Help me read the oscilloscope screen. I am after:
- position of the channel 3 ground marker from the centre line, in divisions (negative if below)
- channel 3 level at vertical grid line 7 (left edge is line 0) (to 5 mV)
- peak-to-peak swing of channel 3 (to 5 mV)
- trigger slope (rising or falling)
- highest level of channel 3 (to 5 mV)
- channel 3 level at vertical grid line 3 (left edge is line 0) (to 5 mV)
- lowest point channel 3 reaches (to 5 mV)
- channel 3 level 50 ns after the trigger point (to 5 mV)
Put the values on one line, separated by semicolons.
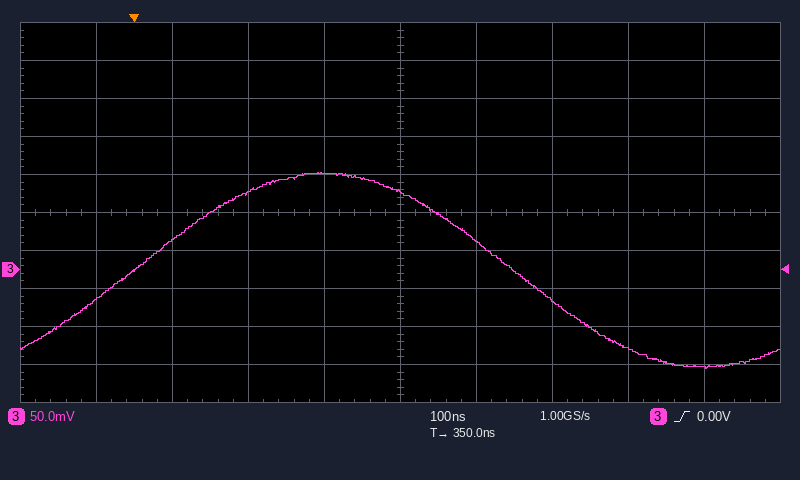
-1.5 div; -40 mV; 260 mV; rising; 130 mV; 100 mV; -130 mV; 40 mV
